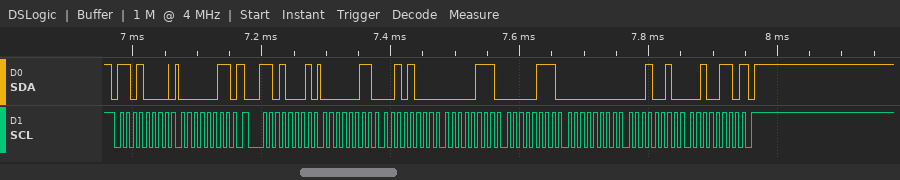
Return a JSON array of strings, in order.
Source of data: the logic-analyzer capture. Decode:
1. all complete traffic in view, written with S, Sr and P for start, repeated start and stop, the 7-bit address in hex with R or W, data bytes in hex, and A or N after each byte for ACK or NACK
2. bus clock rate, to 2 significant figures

["S 68W A 03 A Sr 68R A 03 A 28 A 07 A 07 A 00 A 12 A 26 N P", "100 kHz"]
